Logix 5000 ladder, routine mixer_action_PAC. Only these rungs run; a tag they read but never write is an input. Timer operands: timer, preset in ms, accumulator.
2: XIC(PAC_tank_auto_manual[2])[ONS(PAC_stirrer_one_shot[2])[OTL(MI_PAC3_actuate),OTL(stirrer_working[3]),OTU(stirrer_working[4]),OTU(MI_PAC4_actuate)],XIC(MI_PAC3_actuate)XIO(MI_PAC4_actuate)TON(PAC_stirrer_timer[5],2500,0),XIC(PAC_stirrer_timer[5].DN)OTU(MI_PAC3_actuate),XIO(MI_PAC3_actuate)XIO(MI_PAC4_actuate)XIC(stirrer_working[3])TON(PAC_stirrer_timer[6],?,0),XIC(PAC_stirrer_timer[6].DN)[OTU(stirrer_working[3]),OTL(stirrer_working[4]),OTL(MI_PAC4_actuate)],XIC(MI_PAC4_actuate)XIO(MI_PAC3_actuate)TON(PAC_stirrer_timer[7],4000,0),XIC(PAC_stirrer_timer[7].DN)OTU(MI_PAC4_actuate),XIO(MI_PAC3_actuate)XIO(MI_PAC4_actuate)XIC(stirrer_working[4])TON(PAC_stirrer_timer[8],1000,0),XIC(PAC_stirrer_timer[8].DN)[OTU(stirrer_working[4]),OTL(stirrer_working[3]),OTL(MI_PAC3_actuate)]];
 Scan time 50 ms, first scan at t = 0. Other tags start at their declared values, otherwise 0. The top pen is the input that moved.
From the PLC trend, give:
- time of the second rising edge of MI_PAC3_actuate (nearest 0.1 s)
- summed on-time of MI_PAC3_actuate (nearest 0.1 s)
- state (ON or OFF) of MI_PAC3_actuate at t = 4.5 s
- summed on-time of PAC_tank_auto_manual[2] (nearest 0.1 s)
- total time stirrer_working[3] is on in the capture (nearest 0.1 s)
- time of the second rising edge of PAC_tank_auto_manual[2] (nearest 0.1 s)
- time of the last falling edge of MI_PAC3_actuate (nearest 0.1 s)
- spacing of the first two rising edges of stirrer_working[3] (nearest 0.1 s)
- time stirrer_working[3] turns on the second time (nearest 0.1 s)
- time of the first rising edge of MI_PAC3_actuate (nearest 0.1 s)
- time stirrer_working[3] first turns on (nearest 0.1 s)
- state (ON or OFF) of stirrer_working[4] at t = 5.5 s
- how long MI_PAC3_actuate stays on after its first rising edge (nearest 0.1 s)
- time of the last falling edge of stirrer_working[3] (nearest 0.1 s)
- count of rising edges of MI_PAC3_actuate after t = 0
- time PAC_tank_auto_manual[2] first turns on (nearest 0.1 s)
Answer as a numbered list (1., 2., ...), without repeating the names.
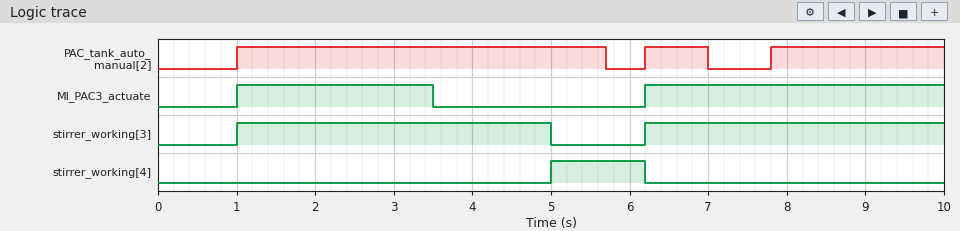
1. 6.2 s
2. 6.3 s
3. OFF
4. 7.7 s
5. 7.8 s
6. 6.2 s
7. 3.5 s
8. 5.2 s
9. 6.2 s
10. 1.0 s
11. 1.0 s
12. ON
13. 2.5 s
14. 5.0 s
15. 2
16. 1.0 s
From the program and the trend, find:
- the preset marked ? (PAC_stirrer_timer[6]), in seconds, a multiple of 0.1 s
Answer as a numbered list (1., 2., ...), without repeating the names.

1. 1.5 s
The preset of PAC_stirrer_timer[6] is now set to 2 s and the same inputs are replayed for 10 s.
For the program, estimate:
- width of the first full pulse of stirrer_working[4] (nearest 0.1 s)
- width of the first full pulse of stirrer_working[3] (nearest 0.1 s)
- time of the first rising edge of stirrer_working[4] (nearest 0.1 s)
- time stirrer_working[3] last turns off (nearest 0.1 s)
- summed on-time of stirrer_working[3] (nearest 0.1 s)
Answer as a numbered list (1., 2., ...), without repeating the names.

1. 0.7 s
2. 4.5 s
3. 5.5 s
4. 5.5 s
5. 8.3 s
